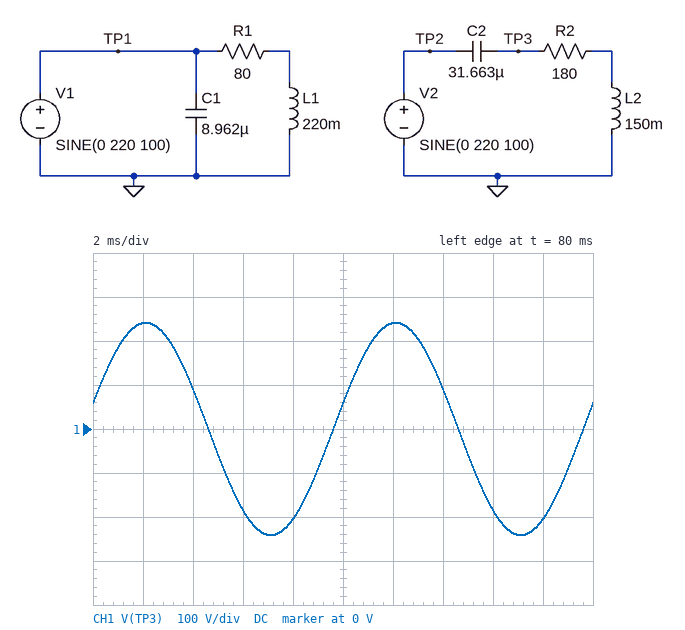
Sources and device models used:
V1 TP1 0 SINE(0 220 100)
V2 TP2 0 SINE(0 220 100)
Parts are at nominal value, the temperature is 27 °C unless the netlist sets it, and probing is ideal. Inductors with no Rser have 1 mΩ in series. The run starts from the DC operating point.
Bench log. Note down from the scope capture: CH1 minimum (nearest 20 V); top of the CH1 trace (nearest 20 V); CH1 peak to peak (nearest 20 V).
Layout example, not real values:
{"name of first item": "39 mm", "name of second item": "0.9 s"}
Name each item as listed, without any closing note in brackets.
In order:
{"CH1 minimum": "-240 V", "top of the CH1 trace": "240 V", "CH1 peak to peak": "480 V"}
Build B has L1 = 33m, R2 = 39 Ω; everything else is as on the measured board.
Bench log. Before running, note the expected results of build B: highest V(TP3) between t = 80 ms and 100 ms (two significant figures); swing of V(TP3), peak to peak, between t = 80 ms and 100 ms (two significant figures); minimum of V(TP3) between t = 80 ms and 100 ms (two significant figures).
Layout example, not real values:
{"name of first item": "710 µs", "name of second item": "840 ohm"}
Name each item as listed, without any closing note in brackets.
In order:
{"highest V(TP3) between t = 80 ms and 100 ms": "380 V", "swing of V(TP3), peak to peak, between t = 80 ms and 100 ms": "760 V", "minimum of V(TP3) between t = 80 ms and 100 ms": "-380 V"}
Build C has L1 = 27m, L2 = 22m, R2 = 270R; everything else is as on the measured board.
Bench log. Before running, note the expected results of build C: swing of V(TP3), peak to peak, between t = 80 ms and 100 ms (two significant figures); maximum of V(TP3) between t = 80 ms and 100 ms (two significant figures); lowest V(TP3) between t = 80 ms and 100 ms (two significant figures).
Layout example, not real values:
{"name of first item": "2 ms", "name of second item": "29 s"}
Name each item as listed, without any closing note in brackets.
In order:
{"swing of V(TP3), peak to peak, between t = 80 ms and 100 ms": "440 V", "maximum of V(TP3) between t = 80 ms and 100 ms": "220 V", "lowest V(TP3) between t = 80 ms and 100 ms": "-220 V"}
